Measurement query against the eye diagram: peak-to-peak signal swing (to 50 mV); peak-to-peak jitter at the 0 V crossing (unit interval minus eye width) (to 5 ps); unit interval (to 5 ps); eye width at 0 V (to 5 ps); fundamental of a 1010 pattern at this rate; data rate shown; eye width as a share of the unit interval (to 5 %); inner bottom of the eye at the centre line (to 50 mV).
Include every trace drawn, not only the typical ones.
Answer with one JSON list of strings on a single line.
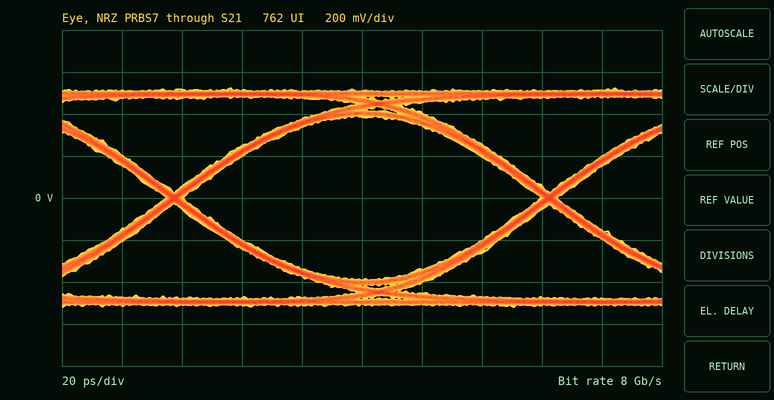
["1.05 V", "5 ps", "125 ps", "120 ps", "4 GHz", "8 Gb/s", "95 %", "-400 mV"]
